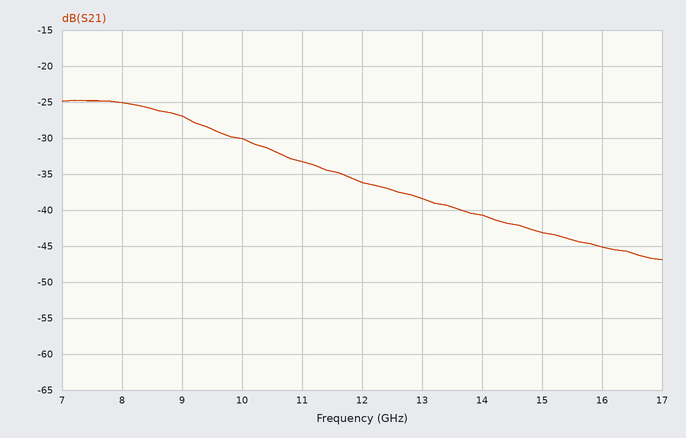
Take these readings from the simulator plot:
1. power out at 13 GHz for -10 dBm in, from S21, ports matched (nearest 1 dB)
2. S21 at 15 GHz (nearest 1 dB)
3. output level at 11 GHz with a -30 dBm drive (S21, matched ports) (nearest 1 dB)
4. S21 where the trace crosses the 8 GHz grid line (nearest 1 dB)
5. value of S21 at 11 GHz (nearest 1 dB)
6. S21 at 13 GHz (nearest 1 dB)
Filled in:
-48 dBm
-43 dB
-63 dBm
-25 dB
-33 dB
-38 dB
